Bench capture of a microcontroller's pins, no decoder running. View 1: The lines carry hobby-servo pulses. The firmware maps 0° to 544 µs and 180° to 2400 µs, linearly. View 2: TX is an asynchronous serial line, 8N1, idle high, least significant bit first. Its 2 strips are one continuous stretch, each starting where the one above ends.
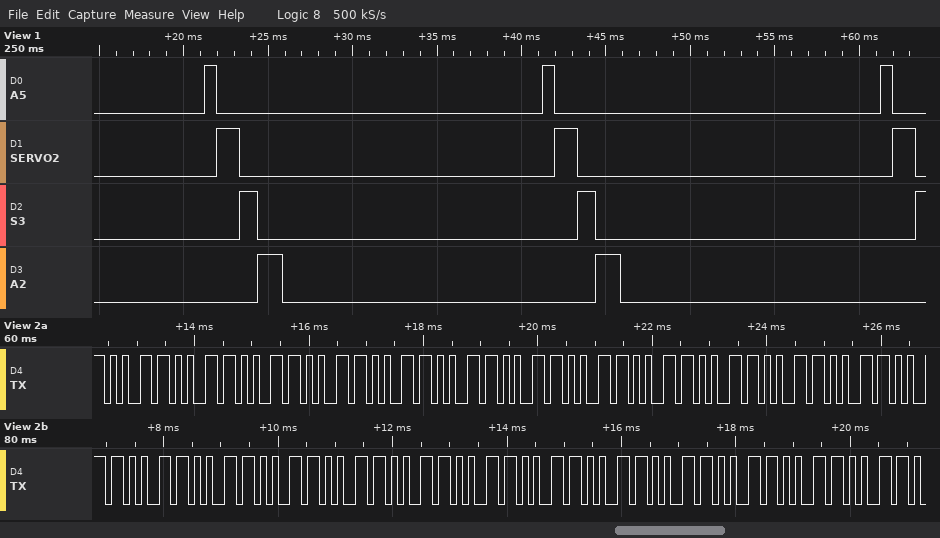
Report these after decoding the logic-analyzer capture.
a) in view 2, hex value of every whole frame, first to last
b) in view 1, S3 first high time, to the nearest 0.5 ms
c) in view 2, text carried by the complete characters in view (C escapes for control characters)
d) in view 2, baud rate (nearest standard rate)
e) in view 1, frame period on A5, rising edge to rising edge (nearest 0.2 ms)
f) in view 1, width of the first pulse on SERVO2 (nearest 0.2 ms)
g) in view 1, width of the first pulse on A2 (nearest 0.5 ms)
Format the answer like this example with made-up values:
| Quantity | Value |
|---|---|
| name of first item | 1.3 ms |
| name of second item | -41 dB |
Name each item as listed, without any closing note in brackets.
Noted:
| Quantity | Value |
|---|---|
| in view 2, hex value of every whole frame, first to last | 65 65 65 65 65 65 65 65 65 65 65 65 65 65 65 65 65 65 65 65 65 65 65 65 65 |
| in view 1, S3 first high time, to the nearest 0.5 ms | 1.0 ms |
| in view 2, text carried by the complete characters in view | "eeeeeeeeeeeeeeeeeeeeeeeee" |
| in view 2, baud rate | 9600 baud |
| in view 1, frame period on A5, rising edge to rising edge | 20.0 ms |
| in view 1, width of the first pulse on SERVO2 | 1.4 ms |
| in view 1, width of the first pulse on A2 | 1.5 ms |
